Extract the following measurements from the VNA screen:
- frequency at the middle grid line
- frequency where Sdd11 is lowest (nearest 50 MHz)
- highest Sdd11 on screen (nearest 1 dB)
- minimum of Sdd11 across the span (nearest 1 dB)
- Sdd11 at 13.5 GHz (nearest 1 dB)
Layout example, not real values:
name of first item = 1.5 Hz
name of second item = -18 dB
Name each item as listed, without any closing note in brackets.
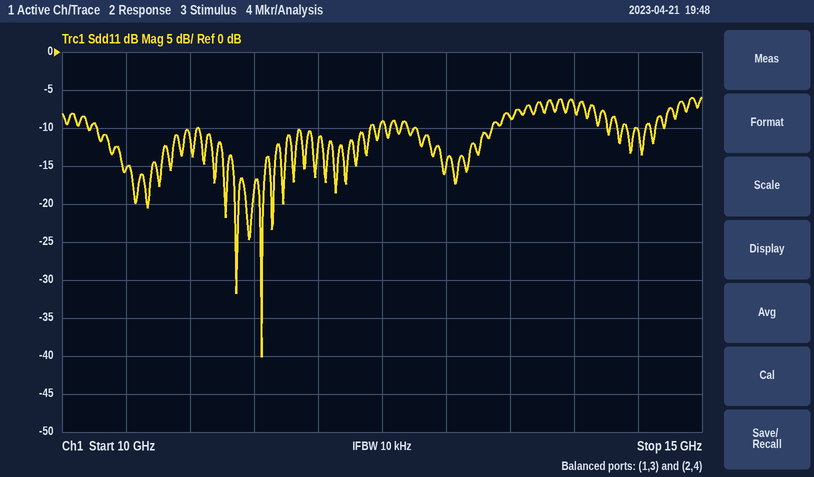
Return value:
frequency at the middle grid line = 12.5 GHz
frequency where Sdd11 is lowest = 11.55 GHz
highest Sdd11 on screen = -6 dB
minimum of Sdd11 across the span = -40 dB
Sdd11 at 13.5 GHz = -9 dB
